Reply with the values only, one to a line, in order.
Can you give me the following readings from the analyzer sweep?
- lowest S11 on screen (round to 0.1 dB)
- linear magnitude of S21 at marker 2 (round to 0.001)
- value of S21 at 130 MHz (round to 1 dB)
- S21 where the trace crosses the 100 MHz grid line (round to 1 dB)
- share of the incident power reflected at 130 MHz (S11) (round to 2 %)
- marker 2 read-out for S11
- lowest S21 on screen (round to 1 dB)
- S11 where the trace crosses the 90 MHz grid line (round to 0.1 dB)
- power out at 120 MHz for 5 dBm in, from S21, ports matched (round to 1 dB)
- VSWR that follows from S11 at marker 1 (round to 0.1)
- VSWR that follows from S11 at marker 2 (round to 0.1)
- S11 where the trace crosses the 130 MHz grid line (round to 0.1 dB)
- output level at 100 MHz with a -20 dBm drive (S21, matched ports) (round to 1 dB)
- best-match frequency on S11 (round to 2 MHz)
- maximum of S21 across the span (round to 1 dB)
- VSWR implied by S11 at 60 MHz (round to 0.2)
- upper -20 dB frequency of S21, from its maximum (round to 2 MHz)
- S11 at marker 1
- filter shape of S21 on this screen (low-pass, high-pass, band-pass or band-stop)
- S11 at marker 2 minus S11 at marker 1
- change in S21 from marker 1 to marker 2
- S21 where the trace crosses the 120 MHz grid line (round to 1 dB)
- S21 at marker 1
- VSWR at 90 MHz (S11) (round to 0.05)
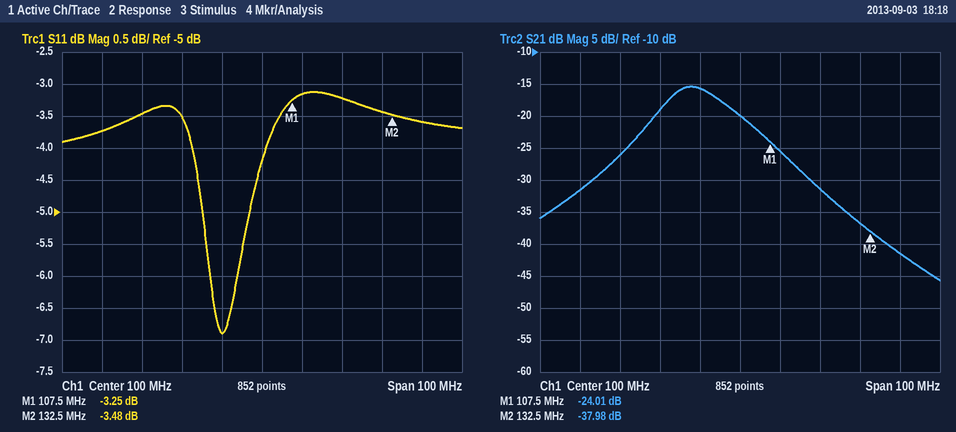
-6.9 dB
0.013
-37 dB
-20 dB
46 %
-3.48 dB
-46 dB
-6.9 dB
-26 dBm
5.4
5.1
-3.4 dB
-40 dBm
90 MHz
-15 dB
4.8
128 MHz
-3.25 dB
band-pass
-0.23 dB
-13.97 dB
-31 dB
-24.01 dB
2.65
